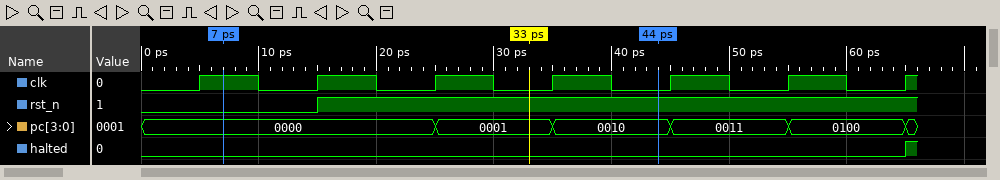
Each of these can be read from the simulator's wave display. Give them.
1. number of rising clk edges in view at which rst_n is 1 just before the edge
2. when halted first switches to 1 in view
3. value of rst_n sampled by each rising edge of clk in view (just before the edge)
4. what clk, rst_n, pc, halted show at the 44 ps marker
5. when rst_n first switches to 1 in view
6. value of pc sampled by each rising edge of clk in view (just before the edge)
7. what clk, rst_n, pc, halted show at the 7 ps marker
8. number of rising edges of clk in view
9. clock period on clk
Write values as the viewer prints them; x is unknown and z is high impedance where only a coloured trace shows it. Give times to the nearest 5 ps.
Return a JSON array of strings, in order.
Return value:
["5", "65 ps", "0 0 1 1 1 1 1", "clk=0, rst_n=1, pc=0010, halted=0", "15 ps", "0000, 0000, 0000, 0001, 0010, 0011, 0100", "clk=1, rst_n=0, pc=0000, halted=0", "7", "10 ps"]
